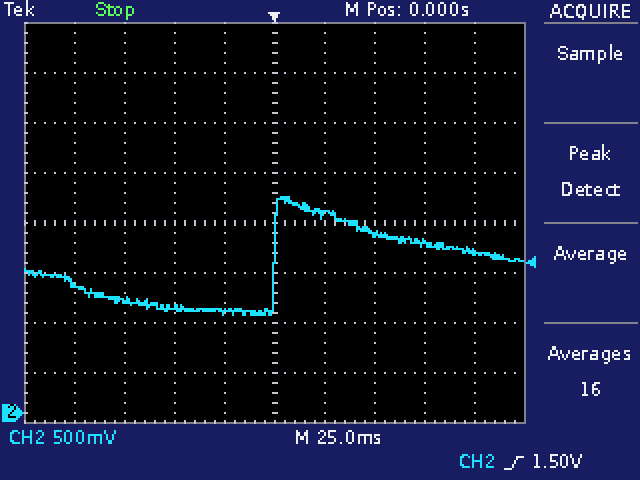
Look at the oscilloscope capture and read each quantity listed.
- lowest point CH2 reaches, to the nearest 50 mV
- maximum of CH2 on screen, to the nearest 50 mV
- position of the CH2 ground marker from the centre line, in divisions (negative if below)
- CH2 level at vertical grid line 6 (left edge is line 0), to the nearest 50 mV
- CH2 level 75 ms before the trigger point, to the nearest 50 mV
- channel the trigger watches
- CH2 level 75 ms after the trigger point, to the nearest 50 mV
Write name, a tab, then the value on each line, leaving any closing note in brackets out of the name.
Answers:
lowest point CH2 reaches, to the nearest 50 mV	1.00 V
maximum of CH2 on screen, to the nearest 50 mV	2.15 V
position of the CH2 ground marker from the centre line, in divisions	-3.8 div
CH2 level at vertical grid line 6 (left edge is line 0), to the nearest 50 mV	2.00 V
CH2 level 75 ms before the trigger point, to the nearest 50 mV	1.15 V
channel the trigger watches	CH2
CH2 level 75 ms after the trigger point, to the nearest 50 mV	1.70 V
